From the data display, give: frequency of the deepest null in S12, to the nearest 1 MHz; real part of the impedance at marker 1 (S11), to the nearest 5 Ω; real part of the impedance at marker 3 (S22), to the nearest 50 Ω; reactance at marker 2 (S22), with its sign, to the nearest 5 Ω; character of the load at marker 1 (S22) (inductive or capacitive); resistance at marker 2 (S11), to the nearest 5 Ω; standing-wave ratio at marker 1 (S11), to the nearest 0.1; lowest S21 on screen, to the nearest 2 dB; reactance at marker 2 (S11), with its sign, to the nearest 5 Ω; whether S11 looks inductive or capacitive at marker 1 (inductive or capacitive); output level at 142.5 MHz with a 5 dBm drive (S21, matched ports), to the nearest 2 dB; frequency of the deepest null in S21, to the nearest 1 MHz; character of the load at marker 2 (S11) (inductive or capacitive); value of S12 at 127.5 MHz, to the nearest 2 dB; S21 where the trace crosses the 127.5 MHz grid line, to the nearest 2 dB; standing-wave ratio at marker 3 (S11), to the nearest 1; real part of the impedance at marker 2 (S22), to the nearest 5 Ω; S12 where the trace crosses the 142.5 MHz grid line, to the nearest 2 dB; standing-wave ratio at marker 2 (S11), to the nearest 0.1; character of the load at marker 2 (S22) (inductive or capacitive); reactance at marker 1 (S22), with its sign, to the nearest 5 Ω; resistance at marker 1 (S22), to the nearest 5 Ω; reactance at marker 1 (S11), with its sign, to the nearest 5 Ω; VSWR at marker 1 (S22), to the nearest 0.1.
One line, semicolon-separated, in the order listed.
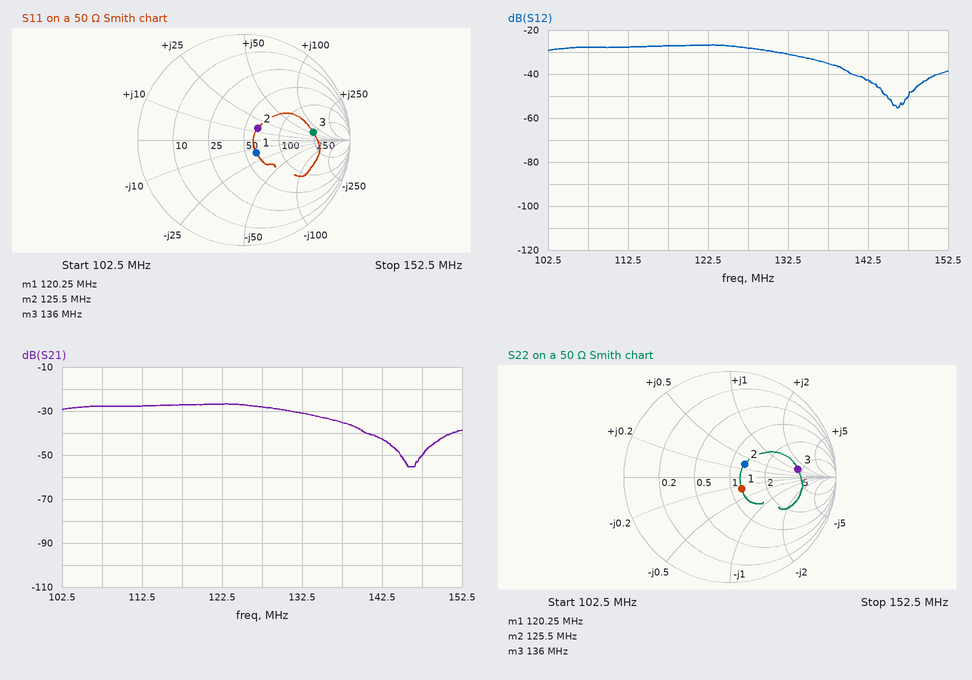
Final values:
146 MHz; 60 Ω; 200 Ω; +15 Ω; capacitive; 65 Ω; 1.4; -56 dB; +15 Ω; capacitive; -38 dBm; 146 MHz; inductive; -28 dB; -28 dB; 5; 65 Ω; -42 dB; 1.4; inductive; -15 Ω; 60 Ω; -15 Ω; 1.4
